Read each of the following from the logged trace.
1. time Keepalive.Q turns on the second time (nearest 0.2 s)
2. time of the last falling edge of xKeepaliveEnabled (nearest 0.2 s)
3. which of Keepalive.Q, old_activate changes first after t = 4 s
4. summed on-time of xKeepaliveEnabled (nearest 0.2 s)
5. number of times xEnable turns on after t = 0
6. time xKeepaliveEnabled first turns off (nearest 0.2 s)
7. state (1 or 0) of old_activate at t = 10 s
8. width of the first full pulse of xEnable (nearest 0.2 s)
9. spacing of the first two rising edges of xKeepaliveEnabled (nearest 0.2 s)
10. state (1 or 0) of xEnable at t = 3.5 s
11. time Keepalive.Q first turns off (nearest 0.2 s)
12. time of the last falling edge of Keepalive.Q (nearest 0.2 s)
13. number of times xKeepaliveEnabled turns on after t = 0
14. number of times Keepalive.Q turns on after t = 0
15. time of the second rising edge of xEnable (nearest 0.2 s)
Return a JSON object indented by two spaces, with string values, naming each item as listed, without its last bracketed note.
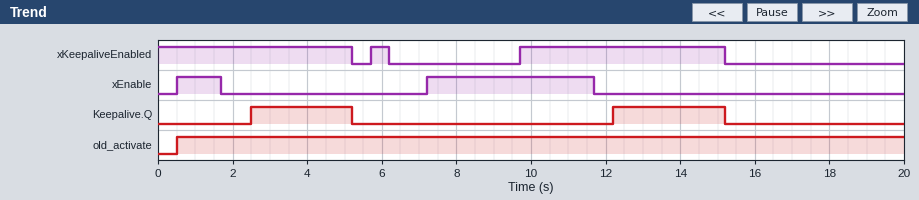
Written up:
{
  "time Keepalive.Q turns on the second time": "12.2 s",
  "time of the last falling edge of xKeepaliveEnabled": "15.2 s",
  "which of Keepalive.Q, old_activate changes first after t = 4 s": "Keepalive.Q",
  "summed on-time of xKeepaliveEnabled": "11.2 s",
  "number of times xEnable turns on after t = 0": "2",
  "time xKeepaliveEnabled first turns off": "5.2 s",
  "state (1 or 0) of old_activate at t = 10 s": "1",
  "width of the first full pulse of xEnable": "1.2 s",
  "spacing of the first two rising edges of xKeepaliveEnabled": "4.0 s",
  "state (1 or 0) of xEnable at t = 3.5 s": "0",
  "time Keepalive.Q first turns off": "5.2 s",
  "time of the last falling edge of Keepalive.Q": "15.2 s",
  "number of times xKeepaliveEnabled turns on after t = 0": "2",
  "number of times Keepalive.Q turns on after t = 0": "2",
  "time of the second rising edge of xEnable": "7.2 s"
}
